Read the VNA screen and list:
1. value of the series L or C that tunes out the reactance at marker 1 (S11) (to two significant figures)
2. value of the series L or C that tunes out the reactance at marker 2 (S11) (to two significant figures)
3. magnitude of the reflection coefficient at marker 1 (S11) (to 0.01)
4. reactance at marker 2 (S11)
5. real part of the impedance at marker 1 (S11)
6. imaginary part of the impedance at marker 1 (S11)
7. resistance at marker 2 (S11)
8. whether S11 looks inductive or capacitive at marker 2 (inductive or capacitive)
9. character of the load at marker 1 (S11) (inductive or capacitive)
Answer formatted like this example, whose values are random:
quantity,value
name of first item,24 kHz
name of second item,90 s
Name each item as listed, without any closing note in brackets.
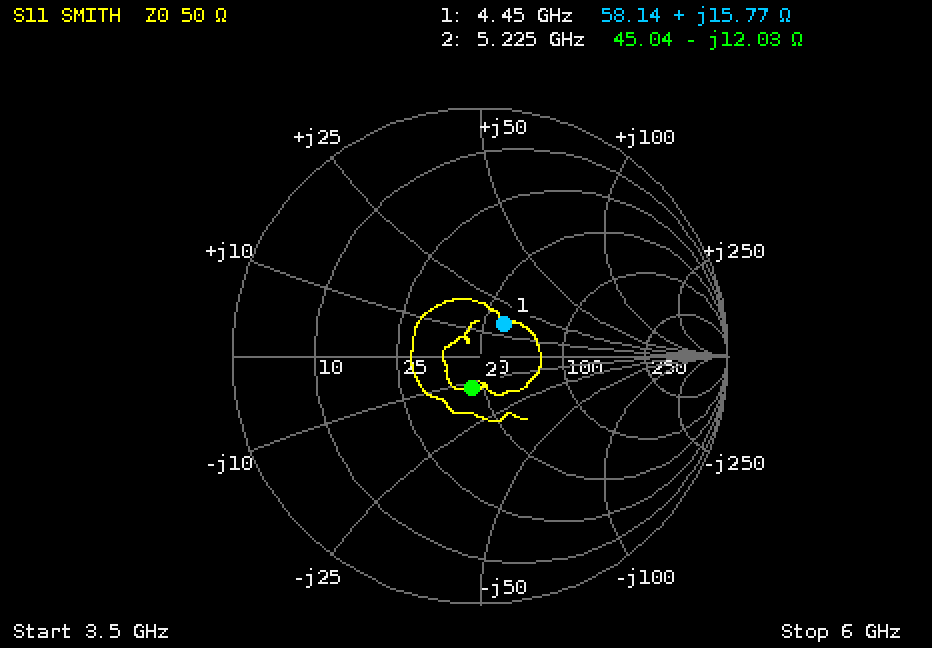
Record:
quantity,value
value of the series L or C that tunes out the reactance at marker 1 (S11),2.3 pF
value of the series L or C that tunes out the reactance at marker 2 (S11),370 pH
magnitude of the reflection coefficient at marker 1 (S11),0.16
reactance at marker 2,-12.03 Ω
real part of the impedance at marker 1,58.14 Ω
imaginary part of the impedance at marker 1,+15.77 Ω
resistance at marker 2,45.04 Ω
whether S11 looks inductive or capacitive at marker 2,capacitive
character of the load at marker 1 (S11),inductive
